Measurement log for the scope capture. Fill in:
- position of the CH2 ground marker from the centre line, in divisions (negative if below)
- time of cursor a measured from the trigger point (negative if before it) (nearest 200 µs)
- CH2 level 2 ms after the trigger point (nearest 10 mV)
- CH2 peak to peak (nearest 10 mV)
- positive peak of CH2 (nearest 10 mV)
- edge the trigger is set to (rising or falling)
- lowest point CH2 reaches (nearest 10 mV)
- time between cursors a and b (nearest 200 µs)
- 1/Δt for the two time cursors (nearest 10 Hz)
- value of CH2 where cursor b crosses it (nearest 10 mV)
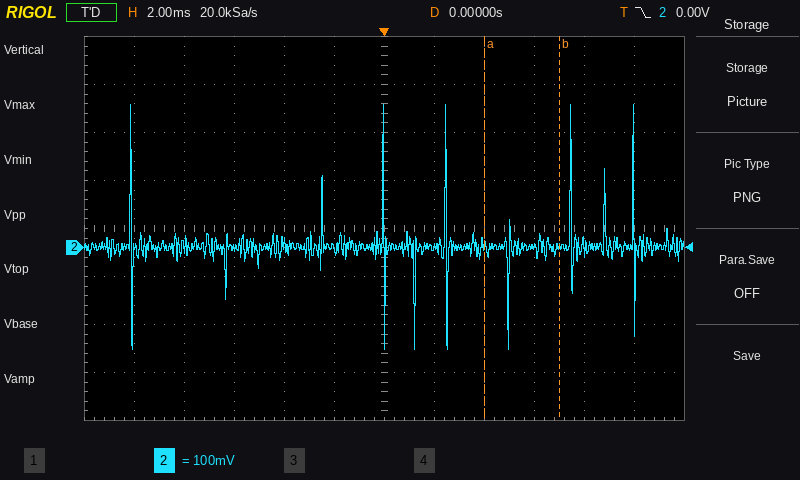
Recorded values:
-0.4 div
+4.0 ms
0 mV
510 mV
300 mV
falling
-210 mV
3.0 ms
330 Hz
0 mV
